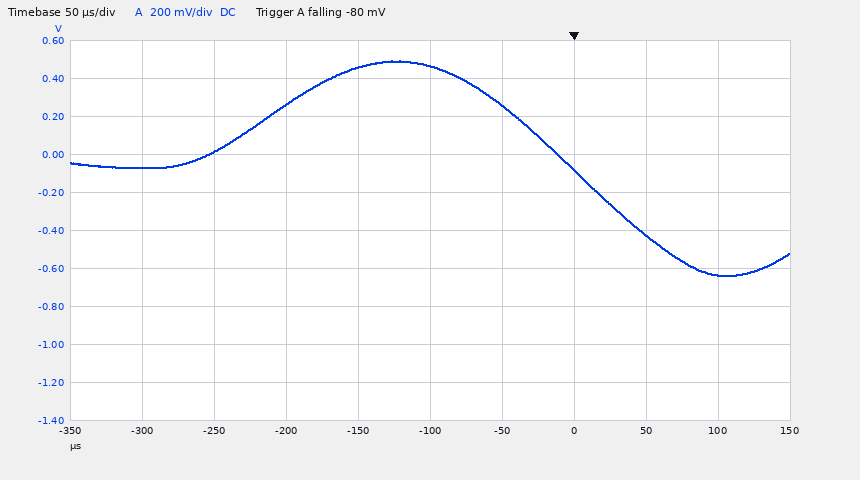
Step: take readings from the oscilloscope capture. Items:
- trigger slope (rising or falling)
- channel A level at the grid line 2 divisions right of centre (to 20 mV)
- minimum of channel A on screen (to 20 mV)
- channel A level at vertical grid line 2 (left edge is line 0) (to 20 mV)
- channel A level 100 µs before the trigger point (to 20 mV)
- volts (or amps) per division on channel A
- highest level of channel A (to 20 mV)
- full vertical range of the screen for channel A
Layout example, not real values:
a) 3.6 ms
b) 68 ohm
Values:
a) falling
b) -80 mV
c) -640 mV
d) 20 mV
e) 460 mV
f) 200 mV
g) 500 mV
h) 2 V
